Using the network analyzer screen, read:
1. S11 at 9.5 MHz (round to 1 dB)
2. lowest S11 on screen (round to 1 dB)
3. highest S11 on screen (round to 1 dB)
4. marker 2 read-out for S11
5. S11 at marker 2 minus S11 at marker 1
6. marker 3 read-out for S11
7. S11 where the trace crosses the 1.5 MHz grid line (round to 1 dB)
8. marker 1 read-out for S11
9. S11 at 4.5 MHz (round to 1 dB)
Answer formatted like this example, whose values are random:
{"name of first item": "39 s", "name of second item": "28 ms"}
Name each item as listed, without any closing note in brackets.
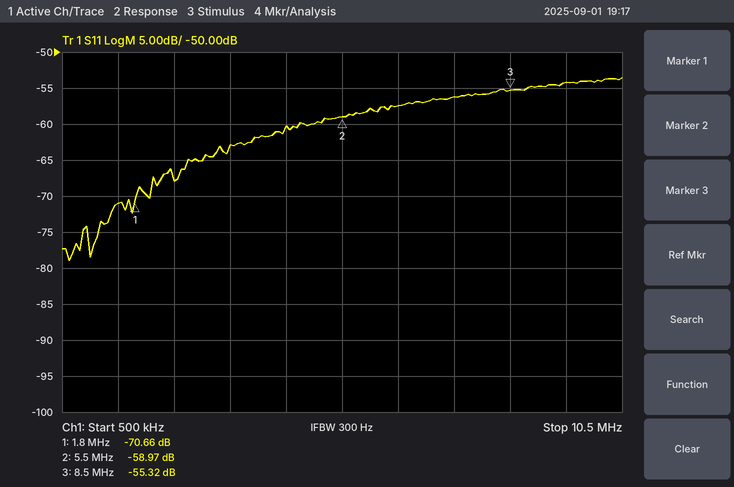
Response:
{"S11 at 9.5 MHz": "-54 dB", "lowest S11 on screen": "-79 dB", "highest S11 on screen": "-54 dB", "marker 2 read-out for S11": "-58.97 dB", "S11 at marker 2 minus S11 at marker 1": "11.69 dB", "marker 3 read-out for S11": "-55.32 dB", "S11 where the trace crosses the 1.5 MHz grid line": "-71 dB", "marker 1 read-out for S11": "-70.66 dB", "S11 at 4.5 MHz": "-60 dB"}
